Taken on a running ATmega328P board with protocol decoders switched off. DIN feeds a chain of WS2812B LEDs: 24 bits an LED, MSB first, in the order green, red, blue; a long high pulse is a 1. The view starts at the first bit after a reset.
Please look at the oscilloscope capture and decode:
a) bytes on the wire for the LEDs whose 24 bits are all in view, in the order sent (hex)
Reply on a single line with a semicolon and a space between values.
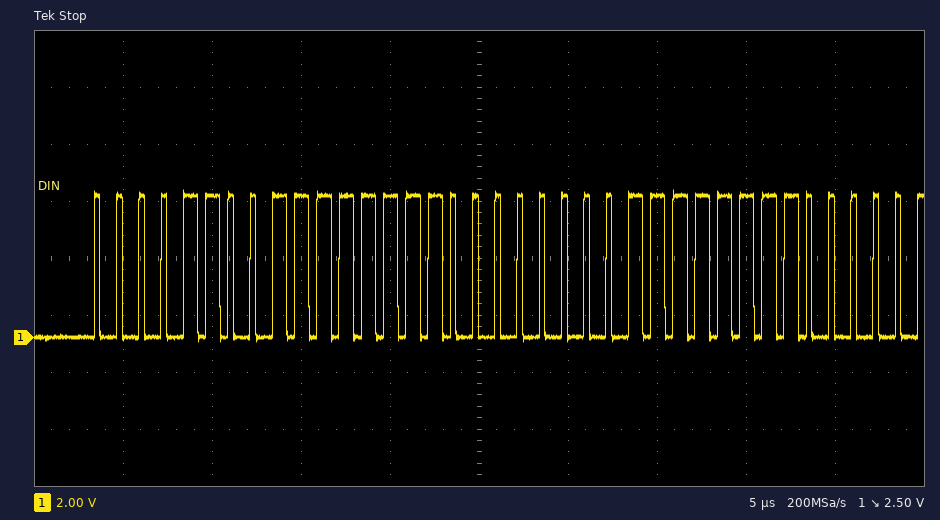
0C FF 00
